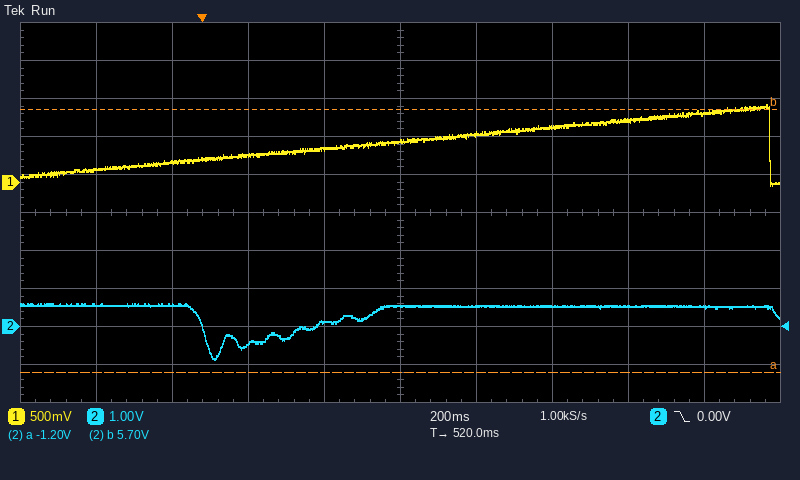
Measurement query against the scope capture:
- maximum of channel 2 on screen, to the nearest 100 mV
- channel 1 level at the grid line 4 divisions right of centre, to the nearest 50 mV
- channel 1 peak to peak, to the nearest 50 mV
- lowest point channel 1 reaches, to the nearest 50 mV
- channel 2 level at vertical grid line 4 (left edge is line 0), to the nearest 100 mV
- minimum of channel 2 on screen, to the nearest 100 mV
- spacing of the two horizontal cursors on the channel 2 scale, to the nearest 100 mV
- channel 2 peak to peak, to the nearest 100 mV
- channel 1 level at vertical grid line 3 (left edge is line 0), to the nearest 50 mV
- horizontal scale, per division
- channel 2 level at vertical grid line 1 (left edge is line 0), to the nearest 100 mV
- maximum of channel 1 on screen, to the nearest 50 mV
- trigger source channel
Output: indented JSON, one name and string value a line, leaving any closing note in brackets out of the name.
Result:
{
  "maximum of channel 2 on screen, to the nearest 100 mV": "600 mV",
  "channel 1 level at the grid line 4 divisions right of centre, to the nearest 50 mV": "900 mV",
  "channel 1 peak to peak, to the nearest 50 mV": "1.05 V",
  "lowest point channel 1 reaches, to the nearest 50 mV": "-50 mV",
  "channel 2 level at vertical grid line 4 (left edge is line 0), to the nearest 100 mV": "100 mV",
  "minimum of channel 2 on screen, to the nearest 100 mV": "-900 mV",
  "spacing of the two horizontal cursors on the channel 2 scale, to the nearest 100 mV": "6.9 V",
  "channel 2 peak to peak, to the nearest 100 mV": "1.5 V",
  "channel 1 level at vertical grid line 3 (left edge is line 0), to the nearest 50 mV": "350 mV",
  "horizontal scale, per division": "200 ms",
  "channel 2 level at vertical grid line 1 (left edge is line 0), to the nearest 100 mV": "600 mV",
  "maximum of channel 1 on screen, to the nearest 50 mV": "1.00 V",
  "trigger source channel": "channel 2"
}
